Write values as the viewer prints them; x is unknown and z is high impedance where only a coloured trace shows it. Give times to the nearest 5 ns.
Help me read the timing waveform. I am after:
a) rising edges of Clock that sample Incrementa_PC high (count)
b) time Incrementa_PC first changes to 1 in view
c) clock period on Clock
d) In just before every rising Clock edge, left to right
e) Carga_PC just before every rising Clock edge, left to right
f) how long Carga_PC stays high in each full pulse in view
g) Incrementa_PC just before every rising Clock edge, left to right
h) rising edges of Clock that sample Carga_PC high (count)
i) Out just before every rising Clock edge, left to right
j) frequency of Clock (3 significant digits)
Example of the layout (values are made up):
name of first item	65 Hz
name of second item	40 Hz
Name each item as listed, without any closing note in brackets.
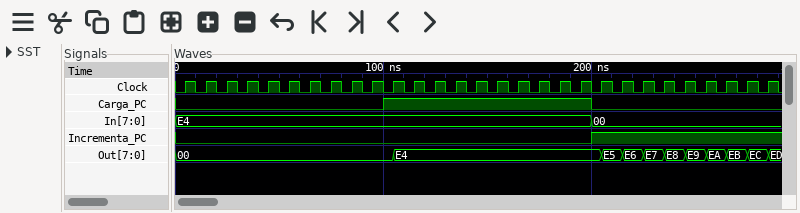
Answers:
rising edges of Clock that sample Incrementa_PC high	9
time Incrementa_PC first changes to 1 in view	200 ns
clock period on Clock	10 ns
In just before every rising Clock edge, left to right	E4, E4, E4, E4, E4, E4, E4, E4, E4, E4, E4, E4, E4, E4, E4, E4, E4, E4, E4, E4, 00, 00, 00, 00, 00, 00, 00, 00, 00
Carga_PC just before every rising Clock edge, left to right	0 0 0 0 0 0 0 0 0 0 1 1 1 1 1 1 1 1 1 1 0 0 0 0 0 0 0 0 0
how long Carga_PC stays high in each full pulse in view	100 ns
Incrementa_PC just before every rising Clock edge, left to right	0 0 0 0 0 0 0 0 0 0 0 0 0 0 0 0 0 0 0 0 1 1 1 1 1 1 1 1 1
rising edges of Clock that sample Carga_PC high	10
Out just before every rising Clock edge, left to right	00, 00, 00, 00, 00, 00, 00, 00, 00, 00, 00, E4, E4, E4, E4, E4, E4, E4, E4, E4, E4, E5, E6, E7, E8, E9, EA, EB, EC
frequency of Clock	100 MHz
